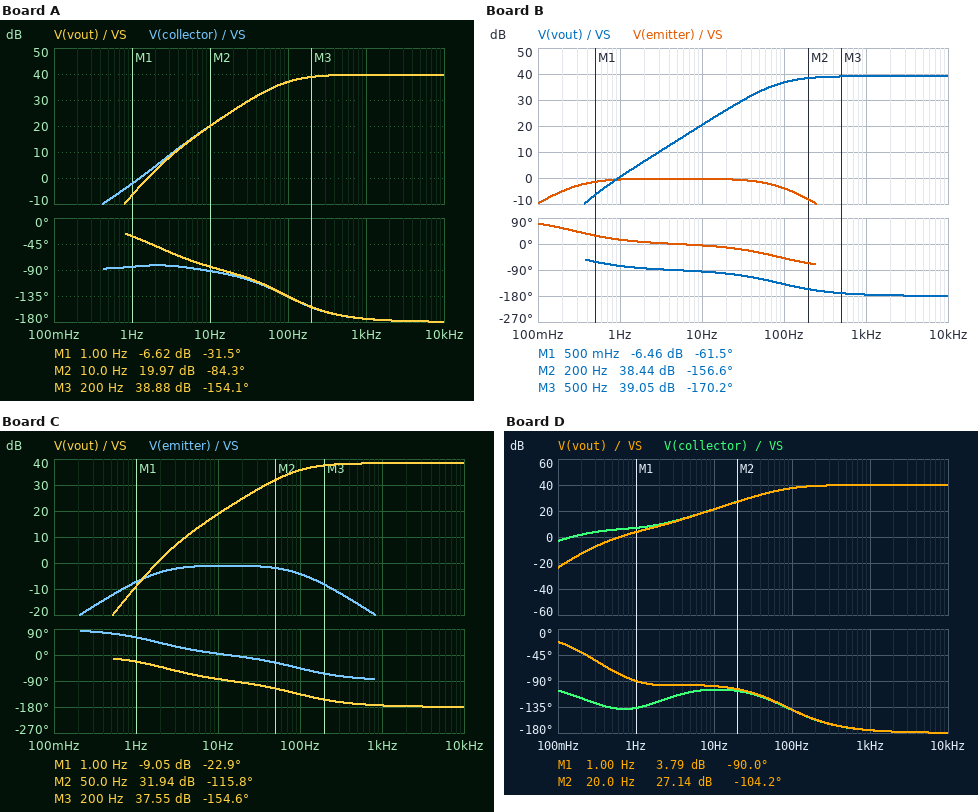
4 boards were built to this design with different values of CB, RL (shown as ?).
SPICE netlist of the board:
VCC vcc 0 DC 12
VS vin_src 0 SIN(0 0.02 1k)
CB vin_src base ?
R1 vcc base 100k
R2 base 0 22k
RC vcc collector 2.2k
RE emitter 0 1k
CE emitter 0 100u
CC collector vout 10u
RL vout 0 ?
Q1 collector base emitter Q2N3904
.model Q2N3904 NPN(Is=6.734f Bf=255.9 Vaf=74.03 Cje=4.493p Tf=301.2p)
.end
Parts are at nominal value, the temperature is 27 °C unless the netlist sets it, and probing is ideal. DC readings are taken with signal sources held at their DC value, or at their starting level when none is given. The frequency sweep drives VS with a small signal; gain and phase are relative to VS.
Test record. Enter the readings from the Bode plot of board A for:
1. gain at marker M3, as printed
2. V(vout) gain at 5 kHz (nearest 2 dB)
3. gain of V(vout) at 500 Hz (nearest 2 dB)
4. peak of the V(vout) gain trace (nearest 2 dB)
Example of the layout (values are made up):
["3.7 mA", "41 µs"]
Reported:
["38.88 dB", "40 dB", "40 dB", "40 dB"]
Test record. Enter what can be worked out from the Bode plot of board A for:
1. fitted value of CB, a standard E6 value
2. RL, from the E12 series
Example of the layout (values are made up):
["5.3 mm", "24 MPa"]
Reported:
["3.3 µF", "12 kΩ"]
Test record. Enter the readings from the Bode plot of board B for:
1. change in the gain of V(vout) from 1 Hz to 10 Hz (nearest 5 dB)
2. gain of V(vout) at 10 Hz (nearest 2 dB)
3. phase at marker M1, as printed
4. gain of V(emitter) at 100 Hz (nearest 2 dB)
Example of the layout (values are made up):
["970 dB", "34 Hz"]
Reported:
["20 dB", "20 dB", "-61.5 deg", "-4 dB"]
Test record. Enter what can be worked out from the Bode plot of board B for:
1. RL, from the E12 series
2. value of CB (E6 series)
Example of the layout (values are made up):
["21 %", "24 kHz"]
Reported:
["8.2 kΩ", "33 µF"]
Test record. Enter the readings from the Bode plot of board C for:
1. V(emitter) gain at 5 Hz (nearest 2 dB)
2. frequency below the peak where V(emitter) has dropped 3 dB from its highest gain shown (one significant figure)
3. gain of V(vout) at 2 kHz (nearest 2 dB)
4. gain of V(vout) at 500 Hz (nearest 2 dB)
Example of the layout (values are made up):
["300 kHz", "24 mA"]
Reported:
["-2 dB", "2 Hz", "38 dB", "38 dB"]
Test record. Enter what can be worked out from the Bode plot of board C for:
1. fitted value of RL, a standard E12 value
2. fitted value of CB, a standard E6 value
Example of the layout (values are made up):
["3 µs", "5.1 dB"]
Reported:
["5.6 kΩ", "4.7 µF"]
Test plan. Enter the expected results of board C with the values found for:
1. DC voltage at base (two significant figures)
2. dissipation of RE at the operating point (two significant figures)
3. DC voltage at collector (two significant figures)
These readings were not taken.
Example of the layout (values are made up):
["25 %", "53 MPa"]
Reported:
["2.1 V", "2.0 mW", "8.9 V"]
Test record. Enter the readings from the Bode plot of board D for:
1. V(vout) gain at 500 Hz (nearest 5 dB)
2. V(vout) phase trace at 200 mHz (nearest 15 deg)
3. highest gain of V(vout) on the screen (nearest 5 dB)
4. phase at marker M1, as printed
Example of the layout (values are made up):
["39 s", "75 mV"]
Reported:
["40 dB", "-45 deg", "40 dB", "-90.0 deg"]
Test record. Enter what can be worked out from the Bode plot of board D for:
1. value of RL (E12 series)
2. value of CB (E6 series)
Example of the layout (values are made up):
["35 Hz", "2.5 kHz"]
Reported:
["15 kΩ", "33 µF"]
